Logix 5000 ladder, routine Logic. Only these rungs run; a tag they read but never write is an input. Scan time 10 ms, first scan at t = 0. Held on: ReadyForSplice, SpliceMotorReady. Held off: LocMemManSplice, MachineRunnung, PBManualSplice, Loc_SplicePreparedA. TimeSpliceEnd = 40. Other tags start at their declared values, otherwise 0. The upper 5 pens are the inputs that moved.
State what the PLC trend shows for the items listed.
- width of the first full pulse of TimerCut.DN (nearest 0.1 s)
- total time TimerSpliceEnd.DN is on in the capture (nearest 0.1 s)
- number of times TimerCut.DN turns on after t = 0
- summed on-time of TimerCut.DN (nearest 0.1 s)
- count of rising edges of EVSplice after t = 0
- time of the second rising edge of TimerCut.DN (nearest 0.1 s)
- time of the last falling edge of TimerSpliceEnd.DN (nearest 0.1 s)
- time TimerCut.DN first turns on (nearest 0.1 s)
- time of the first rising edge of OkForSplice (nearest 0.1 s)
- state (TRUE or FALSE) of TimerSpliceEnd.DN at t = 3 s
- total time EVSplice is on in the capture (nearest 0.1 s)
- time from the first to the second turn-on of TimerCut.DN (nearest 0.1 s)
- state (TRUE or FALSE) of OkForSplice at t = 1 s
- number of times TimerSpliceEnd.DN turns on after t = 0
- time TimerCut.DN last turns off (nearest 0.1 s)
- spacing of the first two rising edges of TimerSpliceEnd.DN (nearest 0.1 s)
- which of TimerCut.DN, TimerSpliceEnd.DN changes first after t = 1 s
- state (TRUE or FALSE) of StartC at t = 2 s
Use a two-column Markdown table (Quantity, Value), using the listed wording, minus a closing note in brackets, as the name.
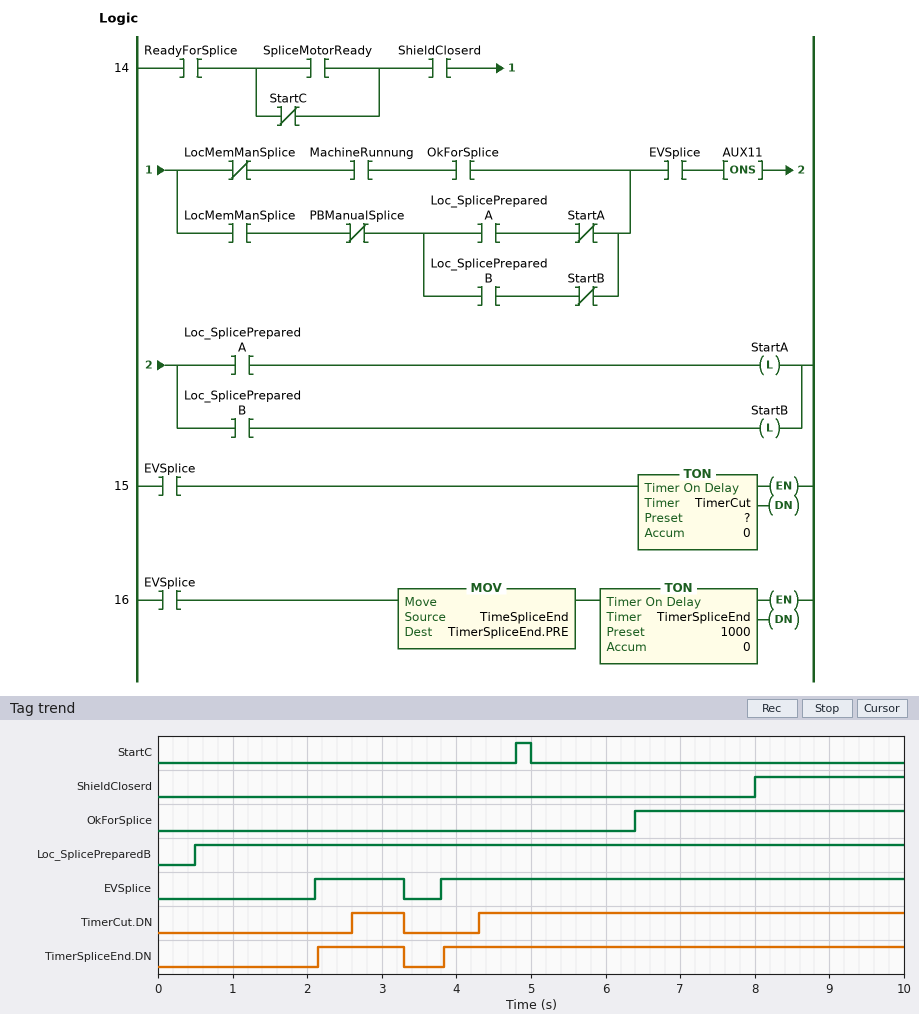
| Quantity | Value |
|---|---|
| width of the first full pulse of TimerCut.DN | 0.7 s |
| total time TimerSpliceEnd.DN is on in the capture | 7.3 s |
| number of times TimerCut.DN turns on after t = 0 | 2 |
| summed on-time of TimerCut.DN | 6.4 s |
| count of rising edges of EVSplice after t = 0 | 2 |
| time of the second rising edge of TimerCut.DN | 4.3 s |
| time of the last falling edge of TimerSpliceEnd.DN | 3.3 s |
| time TimerCut.DN first turns on | 2.6 s |
| time of the first rising edge of OkForSplice | 6.4 s |
| state (TRUE or FALSE) of TimerSpliceEnd.DN at t = 3 s | TRUE |
| total time EVSplice is on in the capture | 7.4 s |
| time from the first to the second turn-on of TimerCut.DN | 1.7 s |
| state (TRUE or FALSE) of OkForSplice at t = 1 s | FALSE |
| number of times TimerSpliceEnd.DN turns on after t = 0 | 2 |
| time TimerCut.DN last turns off | 3.3 s |
| spacing of the first two rising edges of TimerSpliceEnd.DN | 1.7 s |
| which of TimerCut.DN, TimerSpliceEnd.DN changes first after t = 1 s | TimerSpliceEnd.DN |
| state (TRUE or FALSE) of StartC at t = 2 s | FALSE |
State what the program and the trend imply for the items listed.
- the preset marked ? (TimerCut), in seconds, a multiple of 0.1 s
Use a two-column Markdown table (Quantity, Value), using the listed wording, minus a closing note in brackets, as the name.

| Quantity | Value |
|---|---|
| the preset marked ? (TimerCut), in seconds, a multiple of 0.1 s | 0.5 s |
